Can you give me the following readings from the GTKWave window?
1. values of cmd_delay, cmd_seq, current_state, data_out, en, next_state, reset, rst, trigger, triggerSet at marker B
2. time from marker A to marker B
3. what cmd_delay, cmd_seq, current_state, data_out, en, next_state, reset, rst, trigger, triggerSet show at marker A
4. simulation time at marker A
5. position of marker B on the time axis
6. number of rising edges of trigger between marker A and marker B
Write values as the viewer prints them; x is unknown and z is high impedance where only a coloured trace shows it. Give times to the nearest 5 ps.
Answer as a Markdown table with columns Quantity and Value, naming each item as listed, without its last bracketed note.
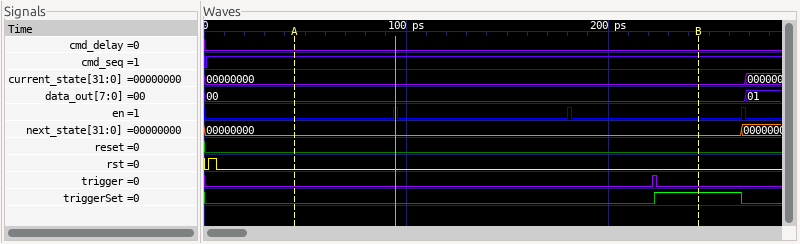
| Quantity | Value |
|---|---|
| values of cmd_delay, cmd_seq, current_state, data_out, en, next_state, reset, rst, trigger, triggerSet at marker B | cmd_delay=0, cmd_seq=1, current_state=00000000, data_out=00, en=0, next_state=00000000, reset=0, rst=0, trigger=0, triggerSet=1 |
| time from marker A to marker B | 200 ps |
| what cmd_delay, cmd_seq, current_state, data_out, en, next_state, reset, rst, trigger, triggerSet show at marker A | cmd_delay=0, cmd_seq=1, current_state=00000000, data_out=00, en=0, next_state=00000000, reset=0, rst=0, trigger=0, triggerSet=0 |
| simulation time at marker A | 45 ps |
| position of marker B on the time axis | 245 ps |
| number of rising edges of trigger between marker A and marker B | 1 |
